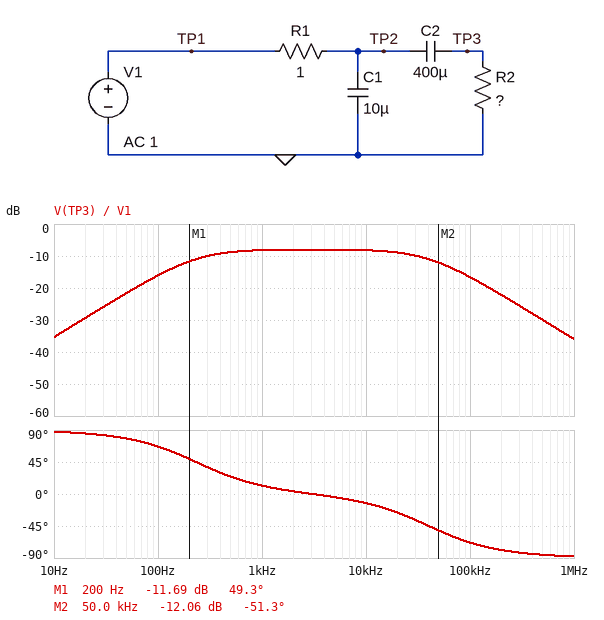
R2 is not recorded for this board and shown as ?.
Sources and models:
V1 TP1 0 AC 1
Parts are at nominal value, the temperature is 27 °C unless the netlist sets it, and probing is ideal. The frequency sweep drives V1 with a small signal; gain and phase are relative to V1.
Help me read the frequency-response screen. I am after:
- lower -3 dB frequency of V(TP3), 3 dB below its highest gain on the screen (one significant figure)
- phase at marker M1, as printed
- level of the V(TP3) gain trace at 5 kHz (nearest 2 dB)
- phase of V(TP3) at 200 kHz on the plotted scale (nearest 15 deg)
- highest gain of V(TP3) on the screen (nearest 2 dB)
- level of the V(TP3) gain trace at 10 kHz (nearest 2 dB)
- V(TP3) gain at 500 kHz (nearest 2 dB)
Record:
200 Hz
49.3 deg
-8 dB
-75 deg
-8 dB
-8 dB
-30 dB
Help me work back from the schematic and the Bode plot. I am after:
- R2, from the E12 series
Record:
0.68 Ω
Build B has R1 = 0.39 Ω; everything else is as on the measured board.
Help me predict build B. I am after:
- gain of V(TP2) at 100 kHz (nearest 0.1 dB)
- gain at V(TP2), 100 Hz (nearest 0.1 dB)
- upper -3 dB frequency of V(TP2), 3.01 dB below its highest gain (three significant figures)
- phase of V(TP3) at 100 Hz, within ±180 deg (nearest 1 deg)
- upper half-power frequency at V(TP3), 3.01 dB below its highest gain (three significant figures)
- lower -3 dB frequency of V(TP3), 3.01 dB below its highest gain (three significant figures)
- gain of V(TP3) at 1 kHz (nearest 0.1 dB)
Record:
-9.3 dB
-0.2 dB
833 Hz
75 deg
65.2 kHz
366 Hz
-4.5 dB
